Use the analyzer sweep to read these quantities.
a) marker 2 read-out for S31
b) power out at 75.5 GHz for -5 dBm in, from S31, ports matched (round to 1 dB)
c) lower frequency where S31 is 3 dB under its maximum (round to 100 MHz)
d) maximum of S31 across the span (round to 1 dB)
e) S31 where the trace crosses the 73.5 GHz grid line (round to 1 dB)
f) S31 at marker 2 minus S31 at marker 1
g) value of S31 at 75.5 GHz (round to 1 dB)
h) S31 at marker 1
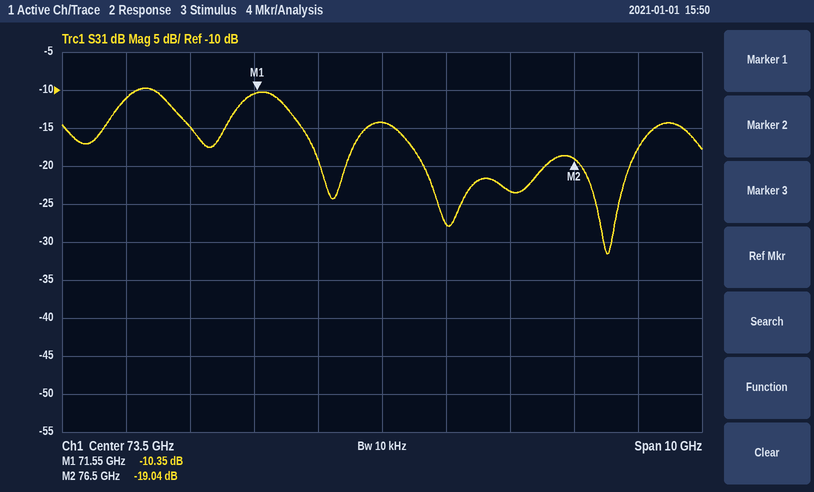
-19.04 dB
-28 dBm
69.3 GHz
-10 dB
-14 dB
-8.69 dB
-23 dB
-10.35 dB
